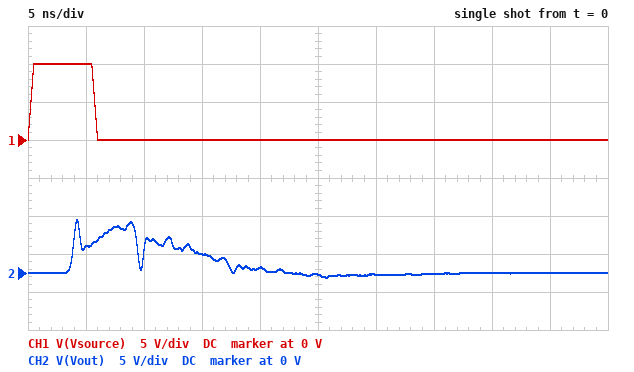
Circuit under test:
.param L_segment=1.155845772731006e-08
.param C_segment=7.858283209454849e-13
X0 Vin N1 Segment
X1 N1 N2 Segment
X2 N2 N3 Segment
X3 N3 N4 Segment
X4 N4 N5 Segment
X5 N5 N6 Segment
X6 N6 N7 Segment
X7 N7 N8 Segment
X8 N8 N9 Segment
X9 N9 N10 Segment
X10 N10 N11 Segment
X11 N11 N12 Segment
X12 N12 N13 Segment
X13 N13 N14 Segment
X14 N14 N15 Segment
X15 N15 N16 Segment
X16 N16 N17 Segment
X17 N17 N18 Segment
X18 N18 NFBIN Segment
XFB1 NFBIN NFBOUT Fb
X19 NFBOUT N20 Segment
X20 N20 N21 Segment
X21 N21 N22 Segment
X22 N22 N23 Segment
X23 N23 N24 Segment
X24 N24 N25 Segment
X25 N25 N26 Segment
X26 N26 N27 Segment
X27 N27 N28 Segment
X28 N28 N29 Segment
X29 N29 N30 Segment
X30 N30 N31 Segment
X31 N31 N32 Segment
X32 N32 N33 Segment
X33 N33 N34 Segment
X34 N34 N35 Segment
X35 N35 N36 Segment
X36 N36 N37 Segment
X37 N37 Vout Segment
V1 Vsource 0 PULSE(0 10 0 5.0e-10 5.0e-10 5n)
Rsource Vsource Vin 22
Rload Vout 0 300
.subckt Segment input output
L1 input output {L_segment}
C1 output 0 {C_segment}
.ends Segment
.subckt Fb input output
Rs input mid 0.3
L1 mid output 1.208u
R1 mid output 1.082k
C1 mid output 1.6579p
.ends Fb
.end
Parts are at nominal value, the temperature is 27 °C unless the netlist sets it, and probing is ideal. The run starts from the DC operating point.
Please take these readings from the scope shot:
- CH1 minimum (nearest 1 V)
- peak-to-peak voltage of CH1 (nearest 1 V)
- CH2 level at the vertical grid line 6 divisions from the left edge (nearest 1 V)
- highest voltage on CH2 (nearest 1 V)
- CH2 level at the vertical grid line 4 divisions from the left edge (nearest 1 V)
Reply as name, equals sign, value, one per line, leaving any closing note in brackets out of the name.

CH1 minimum = 0 V
peak-to-peak voltage of CH1 = 10 V
CH2 level at the vertical grid line 6 divisions from the left edge = 0 V
highest voltage on CH2 = 7 V
CH2 level at the vertical grid line 4 divisions from the left edge = 1 V
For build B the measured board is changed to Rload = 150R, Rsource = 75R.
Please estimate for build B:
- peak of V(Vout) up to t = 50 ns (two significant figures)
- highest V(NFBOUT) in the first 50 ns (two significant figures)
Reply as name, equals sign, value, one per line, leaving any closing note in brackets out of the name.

peak of V(Vout) up to t = 50 ns = 4.0 V
highest V(NFBOUT) in the first 50 ns = 3.8 V
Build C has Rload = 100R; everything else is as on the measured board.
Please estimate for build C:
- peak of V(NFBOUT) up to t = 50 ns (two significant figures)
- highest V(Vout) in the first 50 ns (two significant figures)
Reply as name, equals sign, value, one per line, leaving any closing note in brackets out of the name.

peak of V(NFBOUT) up to t = 50 ns = 4.9 V
highest V(Vout) in the first 50 ns = 4.4 V
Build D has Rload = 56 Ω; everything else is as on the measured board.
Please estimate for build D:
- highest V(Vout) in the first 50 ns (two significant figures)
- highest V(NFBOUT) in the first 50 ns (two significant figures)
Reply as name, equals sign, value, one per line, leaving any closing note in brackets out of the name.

highest V(Vout) in the first 50 ns = 3.1 V
highest V(NFBOUT) in the first 50 ns = 4.9 V
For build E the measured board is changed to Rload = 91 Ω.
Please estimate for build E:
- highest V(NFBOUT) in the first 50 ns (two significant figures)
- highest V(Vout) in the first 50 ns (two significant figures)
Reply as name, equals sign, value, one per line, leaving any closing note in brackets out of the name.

highest V(NFBOUT) in the first 50 ns = 4.9 V
highest V(Vout) in the first 50 ns = 4.2 V
